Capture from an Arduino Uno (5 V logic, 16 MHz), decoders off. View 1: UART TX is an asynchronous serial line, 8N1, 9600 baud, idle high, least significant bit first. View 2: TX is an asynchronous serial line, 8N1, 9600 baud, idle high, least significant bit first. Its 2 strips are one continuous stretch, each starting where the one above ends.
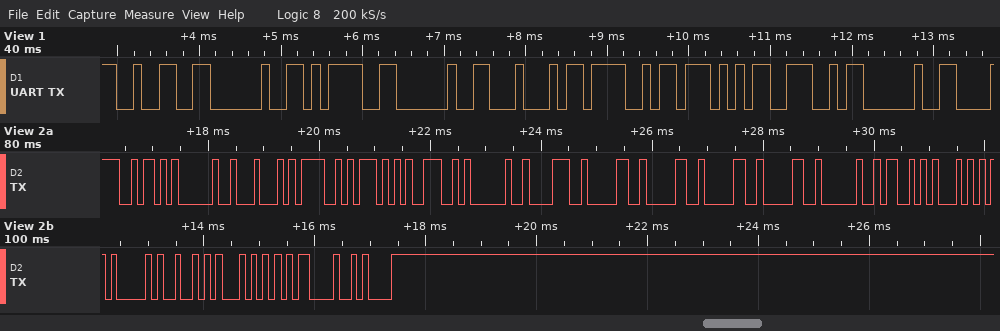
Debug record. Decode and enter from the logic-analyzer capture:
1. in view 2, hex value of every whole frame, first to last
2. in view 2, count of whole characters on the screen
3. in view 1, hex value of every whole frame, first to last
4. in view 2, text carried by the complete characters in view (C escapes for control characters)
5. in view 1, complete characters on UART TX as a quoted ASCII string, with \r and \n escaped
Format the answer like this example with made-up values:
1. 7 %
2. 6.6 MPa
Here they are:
1. 0x5A 0x20 0x44 0x4F 0x57 0x4E 0x20 0x38 0x30 0x30 0x30 0x30 0x20 0x53 0x54 0x41 0x52 0x54 0x0D 0x0A
2. 20
3. 32 20 3D 20 44 4F 57 4E 20
4. "Z DOWN 80000 START\r\n"
5. "2 = DOWN "
